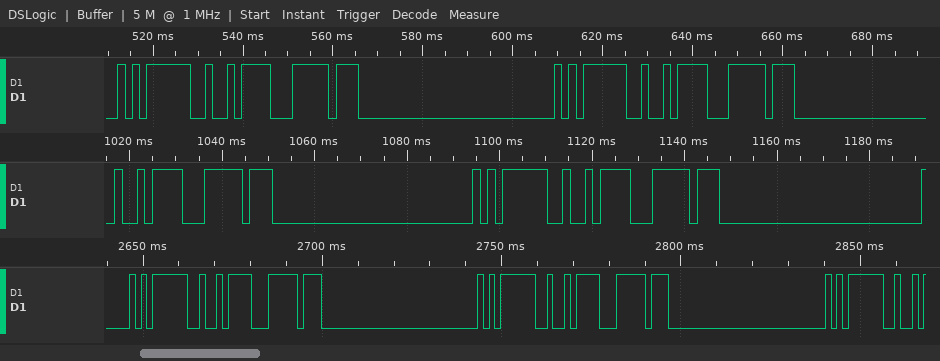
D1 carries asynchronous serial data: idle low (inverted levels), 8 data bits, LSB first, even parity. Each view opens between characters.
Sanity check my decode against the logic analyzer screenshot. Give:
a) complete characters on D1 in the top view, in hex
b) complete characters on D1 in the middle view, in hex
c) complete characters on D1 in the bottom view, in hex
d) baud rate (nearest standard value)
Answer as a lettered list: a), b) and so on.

a) 05, 0B, 10, 05, 0B, 10
b) 0B, 10, 05, 0B, 10
c) 05, 0B, 10, 05, 0B, 10, 05
d) 600 baud
